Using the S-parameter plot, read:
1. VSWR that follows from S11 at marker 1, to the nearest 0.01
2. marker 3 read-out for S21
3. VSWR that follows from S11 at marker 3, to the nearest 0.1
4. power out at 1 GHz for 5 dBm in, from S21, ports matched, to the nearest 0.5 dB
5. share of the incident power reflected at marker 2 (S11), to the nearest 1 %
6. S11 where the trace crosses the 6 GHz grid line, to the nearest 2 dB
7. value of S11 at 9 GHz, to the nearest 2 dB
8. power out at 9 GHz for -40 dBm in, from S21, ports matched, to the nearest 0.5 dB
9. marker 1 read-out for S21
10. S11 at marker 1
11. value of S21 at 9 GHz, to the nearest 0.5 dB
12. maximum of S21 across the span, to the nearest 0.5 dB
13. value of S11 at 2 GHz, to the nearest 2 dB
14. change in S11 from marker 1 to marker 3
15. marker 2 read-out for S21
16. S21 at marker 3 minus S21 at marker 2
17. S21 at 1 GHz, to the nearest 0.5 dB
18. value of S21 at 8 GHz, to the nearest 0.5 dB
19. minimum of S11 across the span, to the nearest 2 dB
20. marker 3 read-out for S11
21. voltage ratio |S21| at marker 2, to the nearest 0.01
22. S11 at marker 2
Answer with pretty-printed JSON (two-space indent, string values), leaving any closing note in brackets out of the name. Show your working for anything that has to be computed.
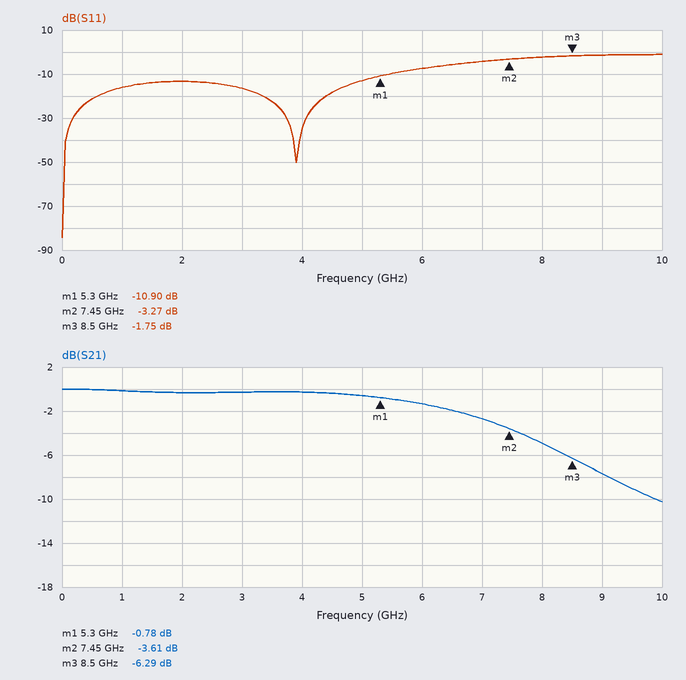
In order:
{
  "VSWR that follows from S11 at marker 1, to the nearest 0.01": "(1 + 0.2851)/(1 − 0.2851) ≈ 1.80",
  "marker 3 read-out for S21": "-6.29 dB",
  "VSWR that follows from S11 at marker 3, to the nearest 0.1": "(1 + 0.8175)/(1 − 0.8175) ≈ 10.0",
  "power out at 1 GHz for 5 dBm in, from S21, ports matched, to the nearest 0.5 dB": "5 dBm + (0.0 dB) = 5.0 dBm",
  "share of the incident power reflected at marker 2 (S11), to the nearest 1 %": "10^(-3.27/10) ≈ 47 %",
  "S11 where the trace crosses the 6 GHz grid line, to the nearest 2 dB": "-8 dB",
  "value of S11 at 9 GHz, to the nearest 2 dB": "-2 dB",
  "power out at 9 GHz for -40 dBm in, from S21, ports matched, to the nearest 0.5 dB": "-40 dBm + (-7.5 dB) = -47.5 dBm",
  "marker 1 read-out for S21": "-0.78 dB",
  "S11 at marker 1": "-10.90 dB",
  "value of S21 at 9 GHz, to the nearest 0.5 dB": "-7.5 dB",
  "maximum of S21 across the span, to the nearest 0.5 dB": "0.0 dB",
  "value of S11 at 2 GHz, to the nearest 2 dB": "-14 dB",
  "change in S11 from marker 1 to marker 3": "-1.75 − (-10.9) = 9.15 dB",
  "marker 2 read-out for S21": "-3.61 dB",
  "S21 at marker 3 minus S21 at marker 2": "-6.29 − (-3.61) = -2.68 dB",
  "S21 at 1 GHz, to the nearest 0.5 dB": "0.0 dB",
  "value of S21 at 8 GHz, to the nearest 0.5 dB": "-5.0 dB",
  "minimum of S11 across the span, to the nearest 2 dB": "-84 dB",
  "marker 3 read-out for S11": "-1.75 dB",
  "voltage ratio |S21| at marker 2, to the nearest 0.01": "10^(-3.61/20) ≈ 0.66",
  "S11 at marker 2": "-3.27 dB"
}
